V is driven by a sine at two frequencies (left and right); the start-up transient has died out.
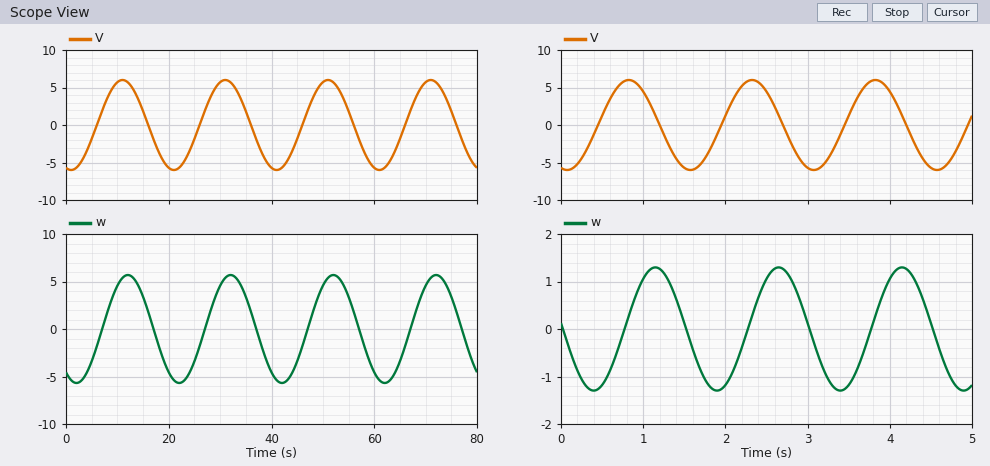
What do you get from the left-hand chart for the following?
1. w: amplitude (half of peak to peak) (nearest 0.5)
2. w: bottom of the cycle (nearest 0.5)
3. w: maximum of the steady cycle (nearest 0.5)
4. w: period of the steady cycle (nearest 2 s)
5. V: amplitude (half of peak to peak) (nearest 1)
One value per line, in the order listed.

5.5
-5.5
5.5
20 s
6
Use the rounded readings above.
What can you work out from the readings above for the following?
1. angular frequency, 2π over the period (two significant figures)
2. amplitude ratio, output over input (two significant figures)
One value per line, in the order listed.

0.31 rad/s
0.92
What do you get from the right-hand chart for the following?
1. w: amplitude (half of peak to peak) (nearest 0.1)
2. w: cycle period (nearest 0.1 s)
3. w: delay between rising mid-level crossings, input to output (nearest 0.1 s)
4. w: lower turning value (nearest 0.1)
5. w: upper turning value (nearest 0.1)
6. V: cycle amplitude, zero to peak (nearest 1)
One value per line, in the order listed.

1.3
1.5 s
0.3 s
-1.3
1.3
6
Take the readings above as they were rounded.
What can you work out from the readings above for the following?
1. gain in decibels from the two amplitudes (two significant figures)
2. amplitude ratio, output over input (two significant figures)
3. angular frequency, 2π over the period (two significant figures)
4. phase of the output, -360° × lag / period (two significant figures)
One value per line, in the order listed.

-13 dB
0.22
4.2 rad/s
-72°
